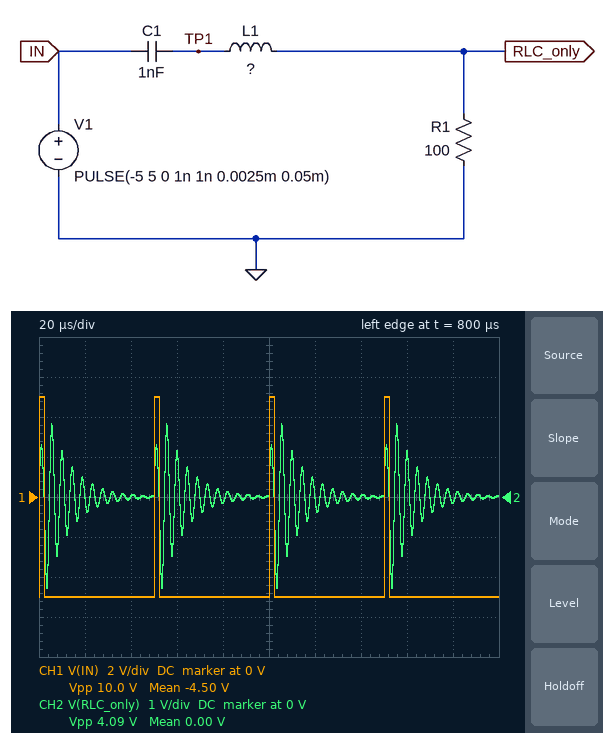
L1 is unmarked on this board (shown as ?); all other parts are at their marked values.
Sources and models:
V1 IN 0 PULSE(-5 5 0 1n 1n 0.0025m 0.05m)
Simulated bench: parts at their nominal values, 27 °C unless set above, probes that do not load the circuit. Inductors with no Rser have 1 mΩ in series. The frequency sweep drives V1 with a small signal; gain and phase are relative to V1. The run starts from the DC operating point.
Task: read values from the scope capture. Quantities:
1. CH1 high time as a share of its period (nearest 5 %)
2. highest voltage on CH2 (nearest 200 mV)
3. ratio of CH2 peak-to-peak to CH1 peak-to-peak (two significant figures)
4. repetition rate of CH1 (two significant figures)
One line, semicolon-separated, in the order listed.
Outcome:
5 %; 1.8 V; 0.41; 20 kHz
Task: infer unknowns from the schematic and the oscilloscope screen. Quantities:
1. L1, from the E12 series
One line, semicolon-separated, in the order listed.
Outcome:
470 µH
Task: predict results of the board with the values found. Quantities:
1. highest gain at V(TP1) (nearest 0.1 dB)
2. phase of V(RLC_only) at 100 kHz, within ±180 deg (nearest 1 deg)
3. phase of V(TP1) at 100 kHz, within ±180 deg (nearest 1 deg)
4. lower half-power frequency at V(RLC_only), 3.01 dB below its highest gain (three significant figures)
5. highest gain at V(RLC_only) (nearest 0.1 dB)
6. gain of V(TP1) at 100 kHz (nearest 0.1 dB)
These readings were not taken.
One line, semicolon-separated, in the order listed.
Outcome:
16.8 dB; 86 deg; 157 deg; 216 kHz; 0 dB; -12.4 dB
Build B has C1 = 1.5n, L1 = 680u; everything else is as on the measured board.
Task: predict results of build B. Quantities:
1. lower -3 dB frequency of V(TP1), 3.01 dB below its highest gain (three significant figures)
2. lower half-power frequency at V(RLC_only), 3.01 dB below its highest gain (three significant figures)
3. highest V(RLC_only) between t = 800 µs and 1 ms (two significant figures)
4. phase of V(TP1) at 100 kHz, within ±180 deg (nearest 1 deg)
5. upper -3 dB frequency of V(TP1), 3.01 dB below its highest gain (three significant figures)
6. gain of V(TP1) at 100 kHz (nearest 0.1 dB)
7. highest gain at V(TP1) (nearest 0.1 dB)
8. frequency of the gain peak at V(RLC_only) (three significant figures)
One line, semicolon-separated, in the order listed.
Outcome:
148 kHz; 146 kHz; 1.8 V; 158 deg; 172 kHz; -3.3 dB; 16.7 dB; 158 kHz
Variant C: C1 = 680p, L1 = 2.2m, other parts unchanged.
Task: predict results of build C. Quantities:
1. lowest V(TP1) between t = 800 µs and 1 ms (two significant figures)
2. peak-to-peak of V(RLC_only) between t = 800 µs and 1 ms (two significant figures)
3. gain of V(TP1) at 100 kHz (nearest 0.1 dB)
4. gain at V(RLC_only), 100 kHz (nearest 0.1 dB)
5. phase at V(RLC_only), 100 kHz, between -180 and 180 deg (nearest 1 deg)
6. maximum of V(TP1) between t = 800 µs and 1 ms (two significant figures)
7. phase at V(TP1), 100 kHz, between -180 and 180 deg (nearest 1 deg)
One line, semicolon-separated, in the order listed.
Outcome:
-12 V; 1.3 V; 3.2 dB; -19.7 dB; 84 deg; 11 V; 170 deg
